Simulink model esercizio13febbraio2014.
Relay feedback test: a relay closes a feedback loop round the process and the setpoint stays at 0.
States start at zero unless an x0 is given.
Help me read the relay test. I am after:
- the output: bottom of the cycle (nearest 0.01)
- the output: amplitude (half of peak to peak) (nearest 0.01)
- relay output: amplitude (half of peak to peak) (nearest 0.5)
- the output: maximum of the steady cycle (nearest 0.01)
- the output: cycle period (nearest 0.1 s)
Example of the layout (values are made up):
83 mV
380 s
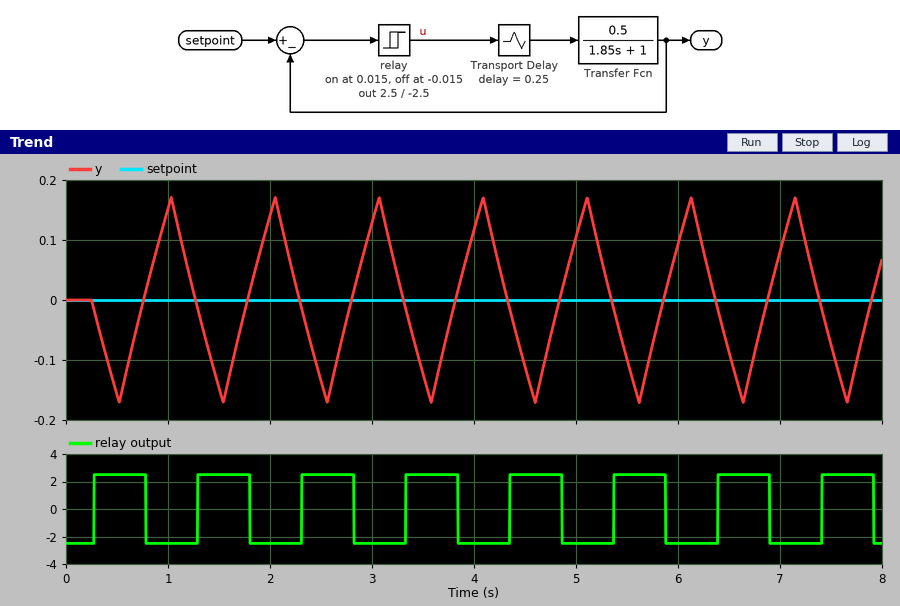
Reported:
-0.17
0.17
2.5
0.17
1.0 s
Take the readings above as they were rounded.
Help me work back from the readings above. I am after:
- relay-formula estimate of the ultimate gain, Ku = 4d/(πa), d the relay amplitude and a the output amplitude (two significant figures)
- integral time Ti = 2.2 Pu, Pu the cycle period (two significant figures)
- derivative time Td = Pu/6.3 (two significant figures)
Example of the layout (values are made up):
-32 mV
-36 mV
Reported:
19
2.2 s
0.16 s
